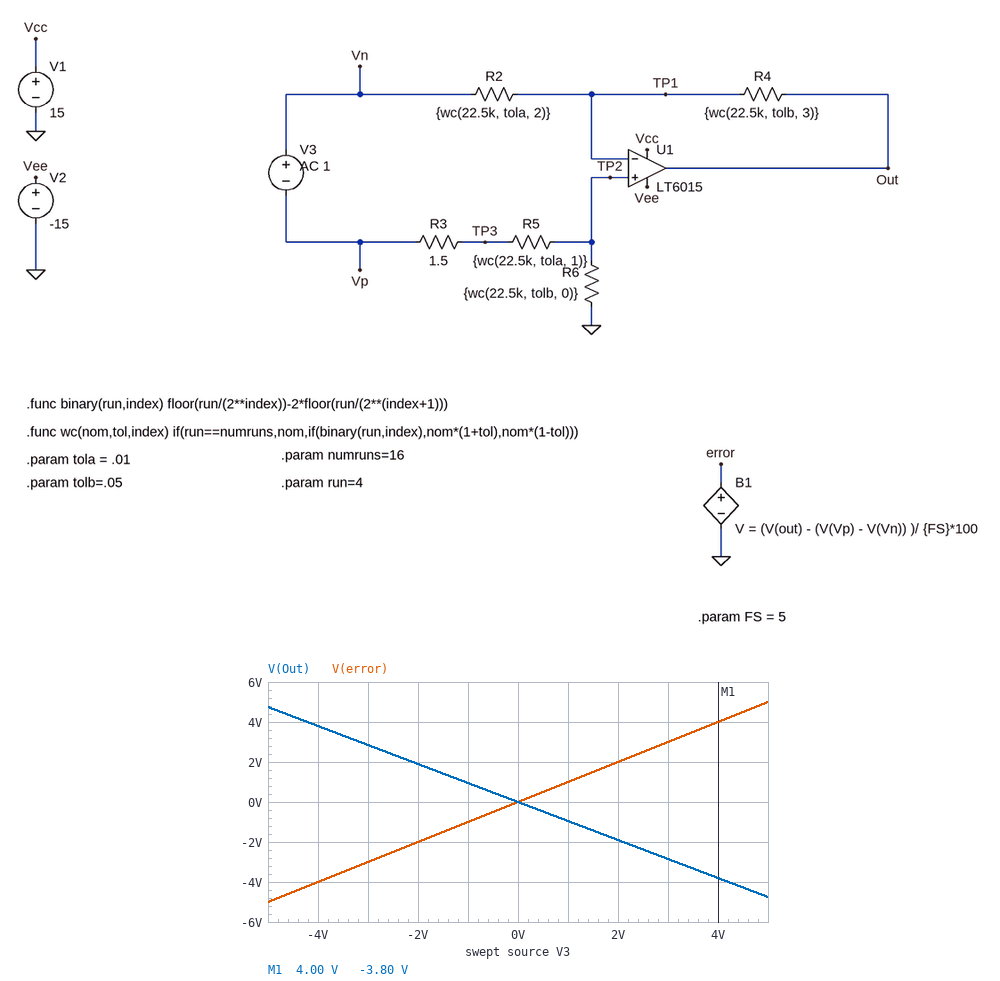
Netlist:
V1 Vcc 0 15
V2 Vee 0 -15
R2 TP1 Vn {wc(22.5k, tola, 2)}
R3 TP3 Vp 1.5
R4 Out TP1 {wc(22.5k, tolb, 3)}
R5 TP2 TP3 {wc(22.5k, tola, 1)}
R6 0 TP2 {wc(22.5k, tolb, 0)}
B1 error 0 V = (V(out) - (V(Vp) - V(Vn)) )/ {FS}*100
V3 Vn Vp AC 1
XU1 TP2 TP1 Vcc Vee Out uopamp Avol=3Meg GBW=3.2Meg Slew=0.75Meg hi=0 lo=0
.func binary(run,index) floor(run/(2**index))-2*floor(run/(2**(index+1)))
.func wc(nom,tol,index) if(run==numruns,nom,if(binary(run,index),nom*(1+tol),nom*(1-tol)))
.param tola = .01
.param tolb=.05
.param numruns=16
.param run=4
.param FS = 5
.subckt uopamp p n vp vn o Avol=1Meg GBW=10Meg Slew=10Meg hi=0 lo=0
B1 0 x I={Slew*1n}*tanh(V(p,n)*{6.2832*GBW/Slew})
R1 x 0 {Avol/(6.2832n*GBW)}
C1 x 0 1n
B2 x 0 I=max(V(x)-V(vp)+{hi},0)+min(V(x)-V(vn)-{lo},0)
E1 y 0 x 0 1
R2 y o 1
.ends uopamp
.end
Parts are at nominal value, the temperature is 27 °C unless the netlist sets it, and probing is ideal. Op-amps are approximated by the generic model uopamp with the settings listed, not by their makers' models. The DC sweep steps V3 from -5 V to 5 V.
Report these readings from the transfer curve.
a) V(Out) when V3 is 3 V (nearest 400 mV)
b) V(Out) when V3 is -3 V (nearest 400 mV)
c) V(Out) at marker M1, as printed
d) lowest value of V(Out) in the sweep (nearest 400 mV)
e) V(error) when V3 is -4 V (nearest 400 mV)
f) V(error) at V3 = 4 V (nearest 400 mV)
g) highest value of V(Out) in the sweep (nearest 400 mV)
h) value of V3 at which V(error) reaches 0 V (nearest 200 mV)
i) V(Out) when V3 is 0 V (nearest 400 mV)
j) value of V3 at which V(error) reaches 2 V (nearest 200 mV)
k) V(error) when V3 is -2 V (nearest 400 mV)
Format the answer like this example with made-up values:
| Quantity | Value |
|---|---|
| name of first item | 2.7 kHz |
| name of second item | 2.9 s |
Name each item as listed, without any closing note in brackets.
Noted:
| Quantity | Value |
|---|---|
| V(Out) when V3 is 3 V | -2.8 V |
| V(Out) when V3 is -3 V | 2.8 V |
| V(Out) at marker M1, as printed | -3.80 V |
| lowest value of V(Out) in the sweep | -4.8 V |
| V(error) when V3 is -4 V | -4.0 V |
| V(error) at V3 = 4 V | 4.0 V |
| highest value of V(Out) in the sweep | 4.8 V |
| value of V3 at which V(error) reaches 0 V | 0 V |
| V(Out) when V3 is 0 V | 0 V |
| value of V3 at which V(error) reaches 2 V | 2.0 V |
| V(error) when V3 is -2 V | -2.0 V |
